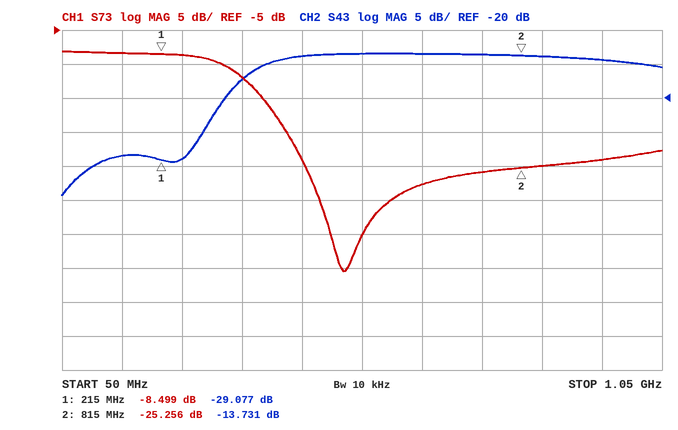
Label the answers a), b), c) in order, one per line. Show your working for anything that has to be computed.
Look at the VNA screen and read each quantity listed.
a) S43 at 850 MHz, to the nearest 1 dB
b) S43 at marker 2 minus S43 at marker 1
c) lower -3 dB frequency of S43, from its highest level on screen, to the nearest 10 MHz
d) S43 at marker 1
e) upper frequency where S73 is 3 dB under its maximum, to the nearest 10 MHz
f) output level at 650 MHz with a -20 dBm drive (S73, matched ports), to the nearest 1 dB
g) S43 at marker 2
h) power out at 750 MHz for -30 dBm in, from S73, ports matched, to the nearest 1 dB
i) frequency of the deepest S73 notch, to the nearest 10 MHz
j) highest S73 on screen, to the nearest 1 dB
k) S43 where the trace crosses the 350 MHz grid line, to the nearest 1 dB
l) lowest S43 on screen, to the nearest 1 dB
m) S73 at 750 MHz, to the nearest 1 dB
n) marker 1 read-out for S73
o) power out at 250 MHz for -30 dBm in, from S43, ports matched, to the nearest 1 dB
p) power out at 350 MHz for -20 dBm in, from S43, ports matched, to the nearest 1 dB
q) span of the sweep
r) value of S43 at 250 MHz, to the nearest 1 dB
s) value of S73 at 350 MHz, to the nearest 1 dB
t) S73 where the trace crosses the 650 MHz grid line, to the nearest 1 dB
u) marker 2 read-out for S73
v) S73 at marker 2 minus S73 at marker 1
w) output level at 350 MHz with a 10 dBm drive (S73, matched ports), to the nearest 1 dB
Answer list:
a) -14 dB
b) -13.731 − (-29.077) = 15.346 dB
c) 360 MHz
d) -29.077 dB
e) 340 MHz
f) -20 dBm + (-28 dB) = -48 dBm
g) -13.731 dB
h) -30 dBm + (-26 dB) = -56 dBm
i) 520 MHz
j) -8 dB
k) -17 dB
l) -34 dB
m) -26 dB
n) -8.499 dB
o) -30 dBm + (-29 dB) = -59 dBm
p) -20 dBm + (-17 dB) = -37 dBm
q) 1 GHz
r) -29 dB
s) -12 dB
t) -28 dB
u) -25.256 dB
v) -25.256 − (-8.499) = -16.757 dB
w) 10 dBm + (-12 dB) = -2 dBm
